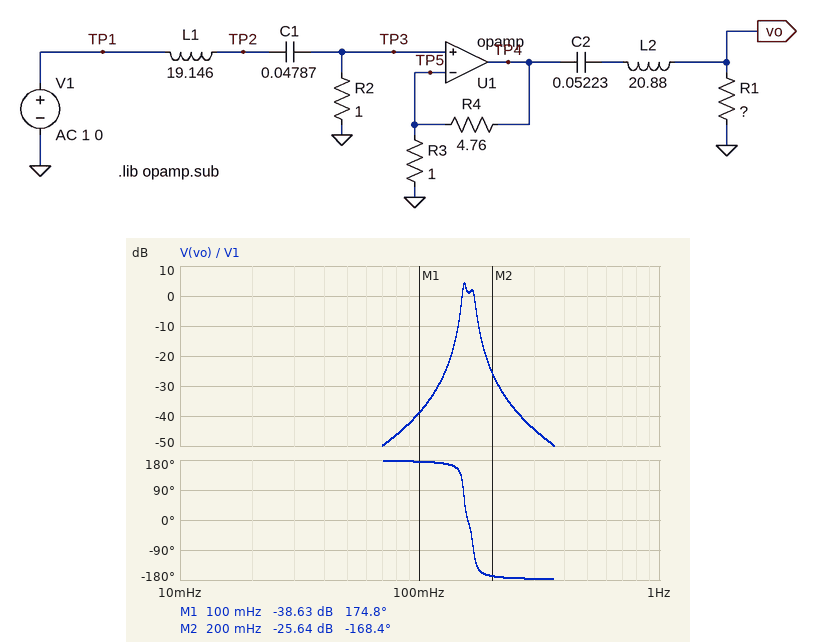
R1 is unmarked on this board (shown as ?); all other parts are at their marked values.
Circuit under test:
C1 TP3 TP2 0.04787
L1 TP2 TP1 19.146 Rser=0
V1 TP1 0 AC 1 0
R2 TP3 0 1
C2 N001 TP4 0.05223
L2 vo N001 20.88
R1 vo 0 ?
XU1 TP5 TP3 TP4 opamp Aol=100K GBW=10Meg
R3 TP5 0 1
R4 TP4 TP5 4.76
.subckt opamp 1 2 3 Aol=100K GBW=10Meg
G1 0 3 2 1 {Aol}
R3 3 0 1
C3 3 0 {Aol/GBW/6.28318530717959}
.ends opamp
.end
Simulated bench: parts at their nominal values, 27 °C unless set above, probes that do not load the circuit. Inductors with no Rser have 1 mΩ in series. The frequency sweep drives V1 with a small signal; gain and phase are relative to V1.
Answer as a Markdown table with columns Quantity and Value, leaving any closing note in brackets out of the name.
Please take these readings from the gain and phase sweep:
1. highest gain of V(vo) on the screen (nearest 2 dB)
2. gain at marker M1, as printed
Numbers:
| Quantity | Value |
|---|---|
| highest gain of V(vo) on the screen | 4 dB |
| gain at marker M1, as printed | -38.63 dB |
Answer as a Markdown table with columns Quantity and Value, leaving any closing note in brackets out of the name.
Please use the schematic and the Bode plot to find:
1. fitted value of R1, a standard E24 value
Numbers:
| Quantity | Value |
|---|---|
| fitted value of R1, a standard E24 value | 0.75 Ω |
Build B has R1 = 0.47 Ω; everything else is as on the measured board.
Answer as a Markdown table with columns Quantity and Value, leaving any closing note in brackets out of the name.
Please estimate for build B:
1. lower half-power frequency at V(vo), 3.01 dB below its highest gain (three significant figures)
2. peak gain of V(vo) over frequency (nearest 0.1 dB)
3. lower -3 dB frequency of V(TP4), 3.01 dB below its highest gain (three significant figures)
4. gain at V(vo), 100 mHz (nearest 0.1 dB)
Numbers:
| Quantity | Value |
|---|---|
| lower half-power frequency at V(vo), 3.01 dB below its highest gain | 151 mHz |
| peak gain of V(vo) over frequency | 4.1 dB |
| lower -3 dB frequency of V(TP4), 3.01 dB below its highest gain | 162 mHz |
| gain at V(vo), 100 mHz | -42.7 dB |
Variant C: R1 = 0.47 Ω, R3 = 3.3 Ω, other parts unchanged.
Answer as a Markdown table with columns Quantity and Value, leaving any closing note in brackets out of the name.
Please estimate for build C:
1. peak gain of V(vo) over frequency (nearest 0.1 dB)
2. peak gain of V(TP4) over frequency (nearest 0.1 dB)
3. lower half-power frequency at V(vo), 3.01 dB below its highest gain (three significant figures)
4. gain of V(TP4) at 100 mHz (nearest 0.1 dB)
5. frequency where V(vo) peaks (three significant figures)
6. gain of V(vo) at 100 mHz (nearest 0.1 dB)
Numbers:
| Quantity | Value |
|---|---|
| peak gain of V(vo) over frequency | -3.4 dB |
| peak gain of V(TP4) over frequency | 7.8 dB |
| lower half-power frequency at V(vo), 3.01 dB below its highest gain | 151 mHz |
| gain of V(TP4) at 100 mHz | -18.8 dB |
| frequency where V(vo) peaks | 153 mHz |
| gain of V(vo) at 100 mHz | -50.1 dB |
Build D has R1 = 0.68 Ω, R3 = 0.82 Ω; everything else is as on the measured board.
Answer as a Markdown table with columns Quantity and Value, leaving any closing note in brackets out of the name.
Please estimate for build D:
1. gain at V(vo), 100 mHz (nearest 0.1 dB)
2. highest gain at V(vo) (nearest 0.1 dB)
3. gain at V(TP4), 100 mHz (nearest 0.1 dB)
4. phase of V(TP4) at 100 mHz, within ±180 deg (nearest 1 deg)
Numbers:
| Quantity | Value |
|---|---|
| gain at V(vo), 100 mHz | -38.0 dB |
| highest gain at V(vo) | 5.6 dB |
| gain at V(TP4), 100 mHz | -9.9 dB |
| phase of V(TP4) at 100 mHz, within ±180 deg | 87 deg |
